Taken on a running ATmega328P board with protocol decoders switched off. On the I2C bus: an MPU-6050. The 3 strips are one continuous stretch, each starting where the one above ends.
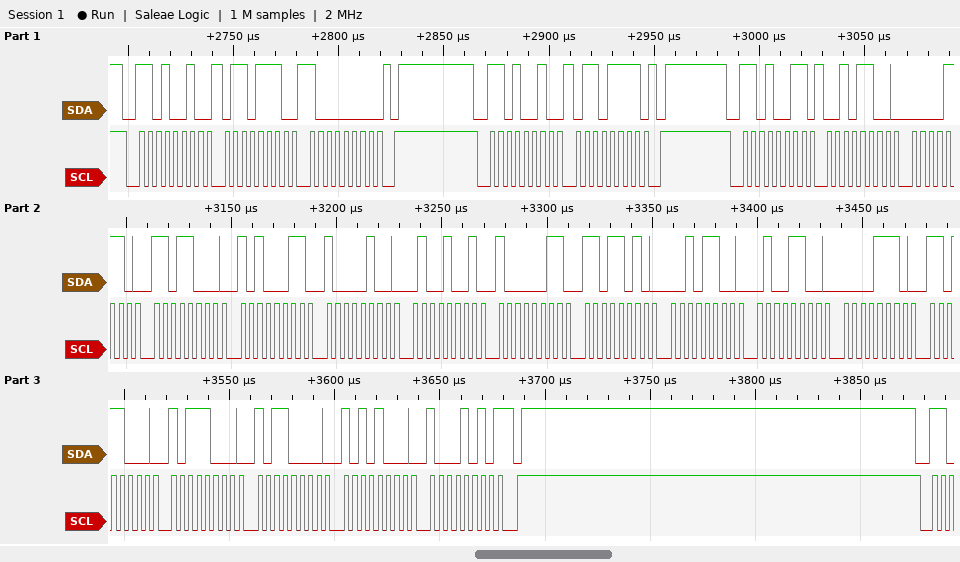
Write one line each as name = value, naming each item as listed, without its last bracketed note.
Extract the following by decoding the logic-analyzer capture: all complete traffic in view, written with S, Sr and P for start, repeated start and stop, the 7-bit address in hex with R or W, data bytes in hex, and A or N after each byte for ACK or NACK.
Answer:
all complete traffic in view, written with S, Sr and P for start, repeated start and stop, the 7-bit address in hex with R or W, data bytes in hex, and A or N after each byte for ACK or NACK = S 69W A 6E A 80 A P S 69W A 6F A P S 69R A 2C A 0E A D8 A A3 A 84 A 49 A 83 A DA A 2C A 4C A 0E A D8 A B8 A B0 A A8 A 8A N P
